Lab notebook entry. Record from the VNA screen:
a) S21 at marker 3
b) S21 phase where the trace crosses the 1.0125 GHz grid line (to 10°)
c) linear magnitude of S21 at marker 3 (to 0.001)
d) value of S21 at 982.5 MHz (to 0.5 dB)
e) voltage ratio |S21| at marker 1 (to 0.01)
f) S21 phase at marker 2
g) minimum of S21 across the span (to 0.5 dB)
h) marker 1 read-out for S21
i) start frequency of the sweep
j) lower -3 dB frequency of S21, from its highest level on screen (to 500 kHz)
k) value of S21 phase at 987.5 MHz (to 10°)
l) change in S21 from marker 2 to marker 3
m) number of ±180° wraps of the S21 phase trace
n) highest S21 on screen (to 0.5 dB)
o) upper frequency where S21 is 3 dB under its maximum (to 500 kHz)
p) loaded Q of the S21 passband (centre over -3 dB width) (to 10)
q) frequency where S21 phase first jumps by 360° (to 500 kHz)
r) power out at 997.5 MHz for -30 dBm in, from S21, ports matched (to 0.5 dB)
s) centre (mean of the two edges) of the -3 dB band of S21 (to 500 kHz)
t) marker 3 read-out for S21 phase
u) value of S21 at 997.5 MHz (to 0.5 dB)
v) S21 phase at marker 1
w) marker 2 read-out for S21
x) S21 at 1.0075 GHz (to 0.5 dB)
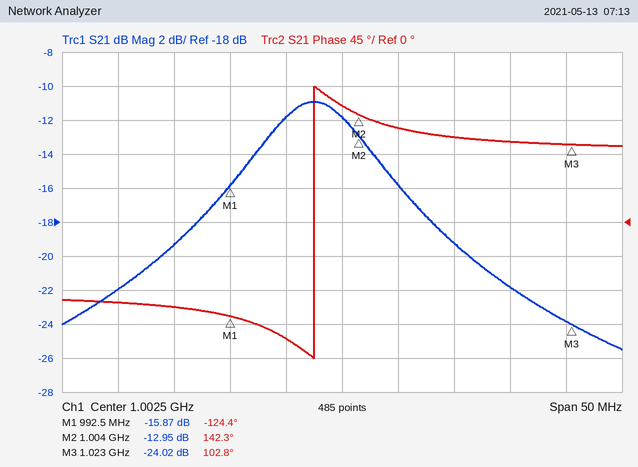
-24.02 dB
110°
0.063
-22.0 dB
0.16
142.3°
-25.5 dB
-15.87 dB
977.5 MHz
995.0 MHz
-110°
-11.07 dB
1
-11.0 dB
1.0050 GHz
100
1.0000 GHz
-42.0 dBm
1.0000 GHz
102.8°
-12.0 dB
-124.4°
-12.95 dB
-16.0 dB
